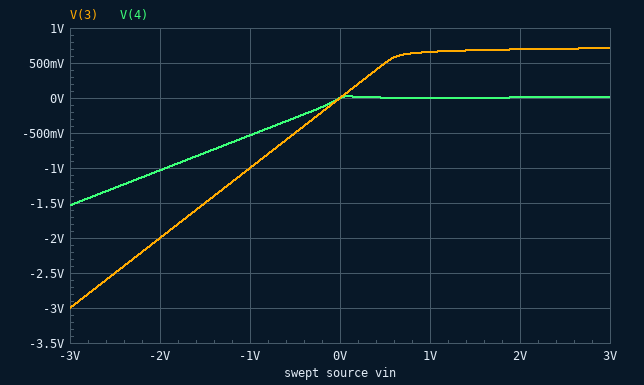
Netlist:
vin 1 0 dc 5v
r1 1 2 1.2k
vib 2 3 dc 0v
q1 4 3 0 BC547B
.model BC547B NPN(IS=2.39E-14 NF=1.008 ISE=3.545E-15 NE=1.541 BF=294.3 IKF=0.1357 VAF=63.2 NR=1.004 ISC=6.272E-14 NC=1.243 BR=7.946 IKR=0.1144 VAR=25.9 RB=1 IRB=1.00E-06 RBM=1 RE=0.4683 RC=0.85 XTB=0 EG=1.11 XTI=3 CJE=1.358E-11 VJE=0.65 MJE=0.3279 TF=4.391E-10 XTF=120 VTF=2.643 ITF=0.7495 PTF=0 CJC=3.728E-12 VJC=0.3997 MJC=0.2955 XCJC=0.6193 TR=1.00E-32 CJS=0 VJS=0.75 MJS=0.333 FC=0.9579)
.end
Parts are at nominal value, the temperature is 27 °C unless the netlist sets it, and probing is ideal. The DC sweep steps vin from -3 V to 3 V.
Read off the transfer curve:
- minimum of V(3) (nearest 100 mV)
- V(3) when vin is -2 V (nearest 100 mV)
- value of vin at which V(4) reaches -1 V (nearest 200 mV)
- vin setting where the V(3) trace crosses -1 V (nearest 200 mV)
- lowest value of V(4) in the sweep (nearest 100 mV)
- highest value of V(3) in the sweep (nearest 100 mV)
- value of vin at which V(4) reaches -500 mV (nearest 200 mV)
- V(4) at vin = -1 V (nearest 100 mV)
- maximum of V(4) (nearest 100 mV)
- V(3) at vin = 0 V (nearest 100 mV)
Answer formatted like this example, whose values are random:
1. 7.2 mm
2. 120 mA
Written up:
1. -3.0 V
2. -2.0 V
3. -2.0 V
4. -1.0 V
5. -1.5 V
6. 700 mV
7. -1.0 V
8. -500 mV
9. 0 V
10. 0 V
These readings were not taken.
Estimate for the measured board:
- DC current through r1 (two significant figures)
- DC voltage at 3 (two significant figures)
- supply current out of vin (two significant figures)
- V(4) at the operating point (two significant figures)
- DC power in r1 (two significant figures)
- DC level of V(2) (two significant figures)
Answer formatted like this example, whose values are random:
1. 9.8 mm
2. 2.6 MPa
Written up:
1. 3.6 mA
2. 730 mV
3. 3.6 mA
4. 9.1 mV
5. 15 mW
6. 730 mV
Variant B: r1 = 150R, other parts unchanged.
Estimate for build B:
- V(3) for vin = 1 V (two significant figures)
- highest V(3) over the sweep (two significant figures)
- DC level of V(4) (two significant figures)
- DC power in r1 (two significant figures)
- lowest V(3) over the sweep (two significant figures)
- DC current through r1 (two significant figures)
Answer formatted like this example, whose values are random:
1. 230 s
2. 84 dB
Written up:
1. 710 mV
2. 790 mV
3. 24 mV
4. 120 mW
5. -3.0 V
6. 28 mA
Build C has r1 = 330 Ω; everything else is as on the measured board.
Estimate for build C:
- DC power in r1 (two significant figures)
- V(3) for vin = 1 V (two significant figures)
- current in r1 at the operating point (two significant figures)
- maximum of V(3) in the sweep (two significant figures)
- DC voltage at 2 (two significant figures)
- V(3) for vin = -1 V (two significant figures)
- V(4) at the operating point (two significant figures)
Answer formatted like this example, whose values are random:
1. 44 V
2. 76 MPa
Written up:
1. 54 mW
2. 690 mV
3. 13 mA
4. 750 mV
5. 780 mV
6. -1.0 V
7. 15 mV
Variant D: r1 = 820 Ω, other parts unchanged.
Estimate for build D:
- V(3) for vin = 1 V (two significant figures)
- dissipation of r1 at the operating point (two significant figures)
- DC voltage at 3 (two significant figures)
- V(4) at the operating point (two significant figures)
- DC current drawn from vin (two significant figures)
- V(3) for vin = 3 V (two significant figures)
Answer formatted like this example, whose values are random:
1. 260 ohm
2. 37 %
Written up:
1. 670 mV
2. 22 mW
3. 740 mV
4. 10 mV
5. 5.2 mA
6. 720 mV
